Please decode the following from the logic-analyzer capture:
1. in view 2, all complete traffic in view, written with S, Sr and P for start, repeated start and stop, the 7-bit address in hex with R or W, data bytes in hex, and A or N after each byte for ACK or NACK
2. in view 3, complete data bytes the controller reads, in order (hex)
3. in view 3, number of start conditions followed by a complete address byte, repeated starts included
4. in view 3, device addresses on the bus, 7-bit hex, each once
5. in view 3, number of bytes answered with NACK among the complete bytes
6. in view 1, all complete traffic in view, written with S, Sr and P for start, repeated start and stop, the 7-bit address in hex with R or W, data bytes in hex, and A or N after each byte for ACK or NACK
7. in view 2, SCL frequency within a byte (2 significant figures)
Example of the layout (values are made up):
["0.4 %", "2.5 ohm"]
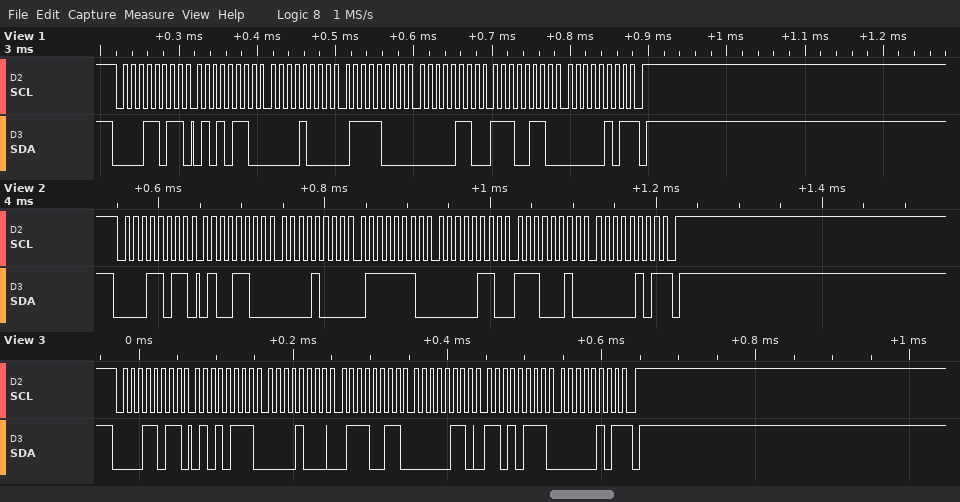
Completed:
["S 0DR A 4C A 08 A 7E A 06 A E2 A 05 N P", "57 08 73 06 D7 05", "1", "0x0D", "1", "S 0DR A 56 A 08 A 78 A 06 A E6 A 05 N P", "100 kHz"]
